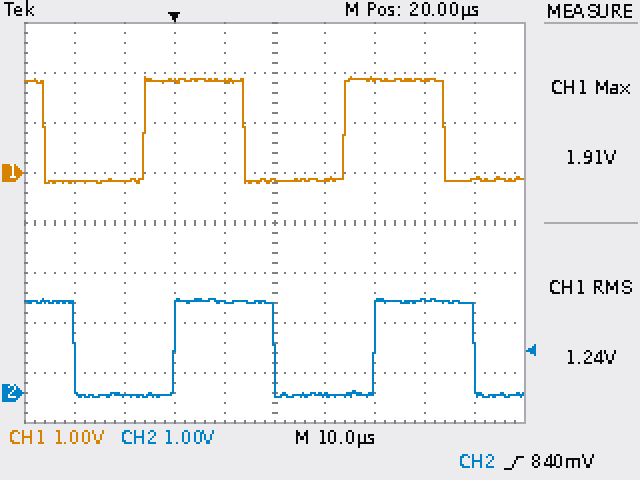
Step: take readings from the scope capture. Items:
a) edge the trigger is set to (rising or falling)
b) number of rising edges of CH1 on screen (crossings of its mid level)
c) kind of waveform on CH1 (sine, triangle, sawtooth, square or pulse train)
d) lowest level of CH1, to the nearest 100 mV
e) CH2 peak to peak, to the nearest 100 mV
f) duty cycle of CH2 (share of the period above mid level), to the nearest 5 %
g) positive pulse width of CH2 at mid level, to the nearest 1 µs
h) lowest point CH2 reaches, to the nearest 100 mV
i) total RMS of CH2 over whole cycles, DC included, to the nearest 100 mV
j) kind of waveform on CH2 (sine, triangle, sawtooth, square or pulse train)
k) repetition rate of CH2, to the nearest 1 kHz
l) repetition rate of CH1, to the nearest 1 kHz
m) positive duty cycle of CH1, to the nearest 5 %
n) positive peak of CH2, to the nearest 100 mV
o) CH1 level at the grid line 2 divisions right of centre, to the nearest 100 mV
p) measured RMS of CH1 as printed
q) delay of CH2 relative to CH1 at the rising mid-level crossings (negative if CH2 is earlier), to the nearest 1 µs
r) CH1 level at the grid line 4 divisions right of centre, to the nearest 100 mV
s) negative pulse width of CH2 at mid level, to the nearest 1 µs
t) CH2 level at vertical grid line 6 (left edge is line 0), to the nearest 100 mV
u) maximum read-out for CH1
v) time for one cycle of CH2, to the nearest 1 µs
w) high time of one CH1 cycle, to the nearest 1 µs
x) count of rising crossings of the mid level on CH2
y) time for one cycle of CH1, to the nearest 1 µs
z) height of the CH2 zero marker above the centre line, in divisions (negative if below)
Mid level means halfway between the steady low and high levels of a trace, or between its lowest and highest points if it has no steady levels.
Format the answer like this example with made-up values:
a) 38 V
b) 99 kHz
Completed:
a) rising
b) 2
c) square
d) -200 mV
e) 2.0 V
f) 50 %
g) 20 µs
h) -100 mV
i) 1.3 V
j) square
k) 25 kHz
l) 25 kHz
m) 50 %
n) 1.9 V
o) 1.9 V
p) 1.24 V
q) +6 µs
r) -100 mV
s) 20 µs
t) 0.0 V
u) 1.91 V
v) 40 µs
w) 20 µs
x) 2
y) 40 µs
z) -3.4 div
